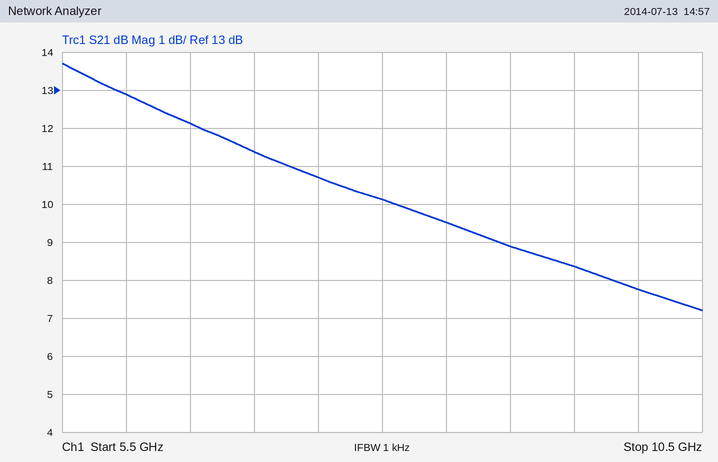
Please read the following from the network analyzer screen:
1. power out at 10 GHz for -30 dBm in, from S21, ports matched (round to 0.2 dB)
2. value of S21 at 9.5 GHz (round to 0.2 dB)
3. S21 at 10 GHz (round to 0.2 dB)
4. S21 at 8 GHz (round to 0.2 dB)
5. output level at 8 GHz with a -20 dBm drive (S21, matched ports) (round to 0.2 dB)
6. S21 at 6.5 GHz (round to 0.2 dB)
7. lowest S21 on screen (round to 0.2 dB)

-22.2 dBm
8.4 dB
7.8 dB
10.2 dB
-9.8 dBm
12.2 dB
7.2 dB
